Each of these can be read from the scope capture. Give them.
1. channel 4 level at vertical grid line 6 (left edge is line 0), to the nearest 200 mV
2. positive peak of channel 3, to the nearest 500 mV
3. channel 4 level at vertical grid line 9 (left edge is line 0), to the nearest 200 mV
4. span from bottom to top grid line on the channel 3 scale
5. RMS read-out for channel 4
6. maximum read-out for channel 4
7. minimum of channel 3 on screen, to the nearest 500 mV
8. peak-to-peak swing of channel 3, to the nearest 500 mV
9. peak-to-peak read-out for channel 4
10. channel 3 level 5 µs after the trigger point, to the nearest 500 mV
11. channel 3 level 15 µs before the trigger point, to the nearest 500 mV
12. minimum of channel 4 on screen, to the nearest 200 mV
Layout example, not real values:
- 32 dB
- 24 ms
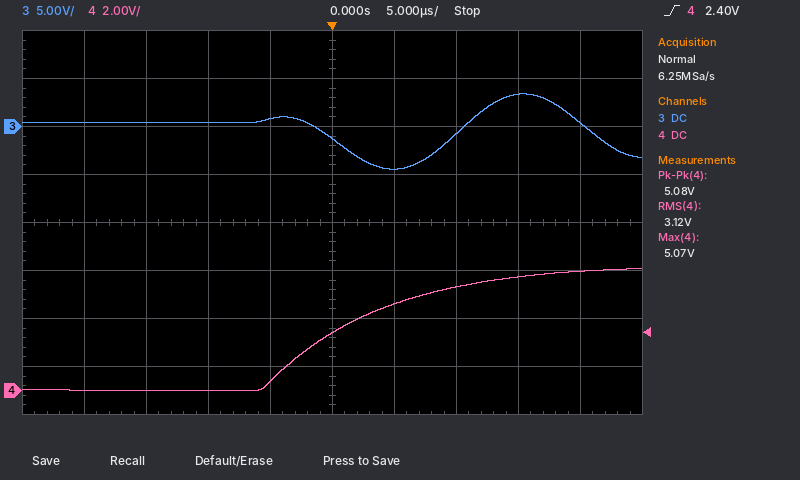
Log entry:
- 3.6 V
- 3.5 V
- 5.0 V
- 40 V
- 3.12 V
- 5.07 V
- -4.5 V
- 8.0 V
- 5.08 V
- -4.5 V
- 500 mV
- 0.0 V
